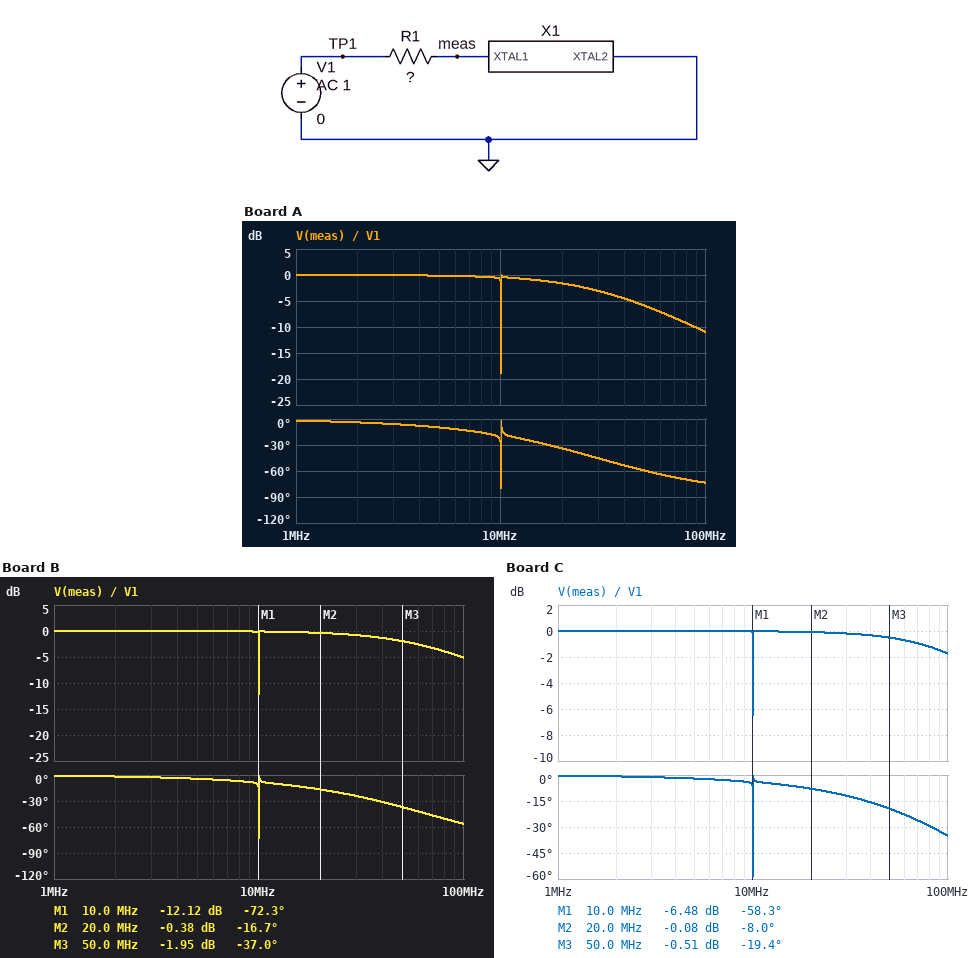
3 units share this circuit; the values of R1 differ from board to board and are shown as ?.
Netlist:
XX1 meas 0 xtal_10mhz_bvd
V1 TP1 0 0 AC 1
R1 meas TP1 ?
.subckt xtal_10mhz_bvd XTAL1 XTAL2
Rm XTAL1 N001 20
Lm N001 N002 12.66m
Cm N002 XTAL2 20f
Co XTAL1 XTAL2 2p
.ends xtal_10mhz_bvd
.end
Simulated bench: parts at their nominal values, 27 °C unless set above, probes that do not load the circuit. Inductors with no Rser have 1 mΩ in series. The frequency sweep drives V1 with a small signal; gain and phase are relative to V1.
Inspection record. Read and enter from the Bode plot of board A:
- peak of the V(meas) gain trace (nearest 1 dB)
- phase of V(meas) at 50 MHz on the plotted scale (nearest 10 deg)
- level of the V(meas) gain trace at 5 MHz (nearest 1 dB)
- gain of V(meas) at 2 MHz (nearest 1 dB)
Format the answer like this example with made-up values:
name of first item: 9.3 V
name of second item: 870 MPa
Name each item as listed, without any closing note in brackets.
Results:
peak of the V(meas) gain trace: 0 dB
phase of V(meas) at 50 MHz on the plotted scale: -60 deg
level of the V(meas) gain trace at 5 MHz: 0 dB
gain of V(meas) at 2 MHz: 0 dB
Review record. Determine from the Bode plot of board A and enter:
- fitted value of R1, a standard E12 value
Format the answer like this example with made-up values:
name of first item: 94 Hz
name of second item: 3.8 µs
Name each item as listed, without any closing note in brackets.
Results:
fitted value of R1, a standard E12 value: 2.7 kΩ
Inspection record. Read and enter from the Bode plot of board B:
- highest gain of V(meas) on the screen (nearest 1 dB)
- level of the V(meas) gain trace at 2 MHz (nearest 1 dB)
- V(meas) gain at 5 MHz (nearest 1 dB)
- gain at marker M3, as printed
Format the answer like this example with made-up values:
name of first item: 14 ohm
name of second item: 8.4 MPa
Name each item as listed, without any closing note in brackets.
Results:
highest gain of V(meas) on the screen: 0 dB
level of the V(meas) gain trace at 2 MHz: 0 dB
V(meas) gain at 5 MHz: 0 dB
gain at marker M3, as printed: -1.95 dB
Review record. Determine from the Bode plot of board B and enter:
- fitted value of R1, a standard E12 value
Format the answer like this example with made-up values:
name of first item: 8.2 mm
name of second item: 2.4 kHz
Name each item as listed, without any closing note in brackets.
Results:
fitted value of R1, a standard E12 value: 1.2 kΩ
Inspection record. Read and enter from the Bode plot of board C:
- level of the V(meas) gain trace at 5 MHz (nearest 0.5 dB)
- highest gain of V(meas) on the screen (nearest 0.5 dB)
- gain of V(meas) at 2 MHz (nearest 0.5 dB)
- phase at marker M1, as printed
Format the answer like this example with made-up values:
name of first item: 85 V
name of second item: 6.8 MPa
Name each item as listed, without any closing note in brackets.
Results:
level of the V(meas) gain trace at 5 MHz: 0 dB
highest gain of V(meas) on the screen: 0 dB
gain of V(meas) at 2 MHz: 0 dB
phase at marker M1, as printed: -58.3 deg
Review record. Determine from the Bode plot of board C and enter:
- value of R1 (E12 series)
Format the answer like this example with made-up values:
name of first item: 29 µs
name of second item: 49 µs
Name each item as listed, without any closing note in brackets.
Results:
value of R1: 560 Ω
